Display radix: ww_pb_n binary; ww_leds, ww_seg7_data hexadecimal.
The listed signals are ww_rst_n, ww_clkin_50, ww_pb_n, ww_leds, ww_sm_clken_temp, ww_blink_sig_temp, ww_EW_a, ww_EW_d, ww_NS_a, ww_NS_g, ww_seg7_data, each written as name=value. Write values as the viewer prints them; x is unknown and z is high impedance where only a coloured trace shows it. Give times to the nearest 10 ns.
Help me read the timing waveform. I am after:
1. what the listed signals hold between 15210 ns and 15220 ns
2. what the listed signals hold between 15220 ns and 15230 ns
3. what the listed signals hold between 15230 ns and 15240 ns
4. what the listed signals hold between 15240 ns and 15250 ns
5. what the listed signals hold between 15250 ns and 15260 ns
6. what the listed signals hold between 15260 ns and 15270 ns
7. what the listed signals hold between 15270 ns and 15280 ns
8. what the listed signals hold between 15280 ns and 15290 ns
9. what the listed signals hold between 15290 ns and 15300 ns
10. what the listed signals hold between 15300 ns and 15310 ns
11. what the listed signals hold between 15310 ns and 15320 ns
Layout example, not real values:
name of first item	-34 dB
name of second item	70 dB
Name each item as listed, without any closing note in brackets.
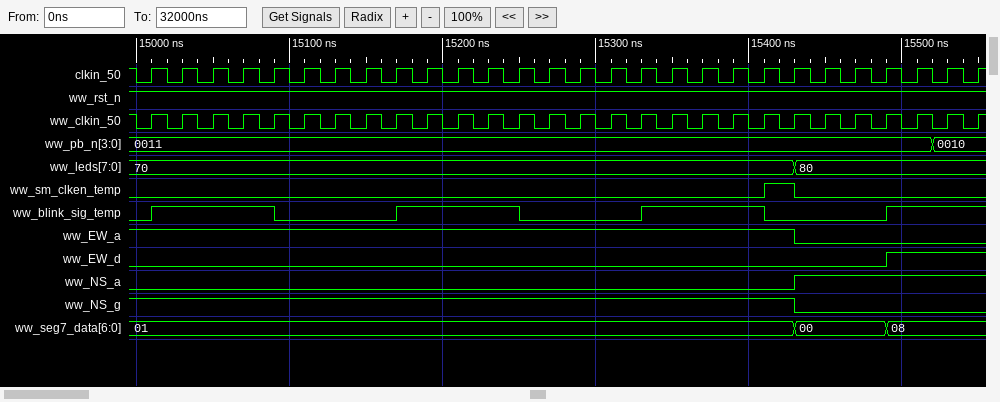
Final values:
what the listed signals hold between 15210 ns and 15220 ns	ww_rst_n=1, ww_clkin_50=1, ww_pb_n=0011, ww_leds=70, ww_sm_clken_temp=0, ww_blink_sig_temp=1, ww_EW_a=1, ww_EW_d=0, ww_NS_a=0, ww_NS_g=1, ww_seg7_data=01
what the listed signals hold between 15220 ns and 15230 ns	ww_rst_n=1, ww_clkin_50=0, ww_pb_n=0011, ww_leds=70, ww_sm_clken_temp=0, ww_blink_sig_temp=1, ww_EW_a=1, ww_EW_d=0, ww_NS_a=0, ww_NS_g=1, ww_seg7_data=01
what the listed signals hold between 15230 ns and 15240 ns	ww_rst_n=1, ww_clkin_50=1, ww_pb_n=0011, ww_leds=70, ww_sm_clken_temp=0, ww_blink_sig_temp=1, ww_EW_a=1, ww_EW_d=0, ww_NS_a=0, ww_NS_g=1, ww_seg7_data=01
what the listed signals hold between 15240 ns and 15250 ns	ww_rst_n=1, ww_clkin_50=0, ww_pb_n=0011, ww_leds=70, ww_sm_clken_temp=0, ww_blink_sig_temp=1, ww_EW_a=1, ww_EW_d=0, ww_NS_a=0, ww_NS_g=1, ww_seg7_data=01
what the listed signals hold between 15250 ns and 15260 ns	ww_rst_n=1, ww_clkin_50=1, ww_pb_n=0011, ww_leds=70, ww_sm_clken_temp=0, ww_blink_sig_temp=0, ww_EW_a=1, ww_EW_d=0, ww_NS_a=0, ww_NS_g=1, ww_seg7_data=01
what the listed signals hold between 15260 ns and 15270 ns	ww_rst_n=1, ww_clkin_50=0, ww_pb_n=0011, ww_leds=70, ww_sm_clken_temp=0, ww_blink_sig_temp=0, ww_EW_a=1, ww_EW_d=0, ww_NS_a=0, ww_NS_g=1, ww_seg7_data=01
what the listed signals hold between 15270 ns and 15280 ns	ww_rst_n=1, ww_clkin_50=1, ww_pb_n=0011, ww_leds=70, ww_sm_clken_temp=0, ww_blink_sig_temp=0, ww_EW_a=1, ww_EW_d=0, ww_NS_a=0, ww_NS_g=1, ww_seg7_data=01
what the listed signals hold between 15280 ns and 15290 ns	ww_rst_n=1, ww_clkin_50=0, ww_pb_n=0011, ww_leds=70, ww_sm_clken_temp=0, ww_blink_sig_temp=0, ww_EW_a=1, ww_EW_d=0, ww_NS_a=0, ww_NS_g=1, ww_seg7_data=01
what the listed signals hold between 15290 ns and 15300 ns	ww_rst_n=1, ww_clkin_50=1, ww_pb_n=0011, ww_leds=70, ww_sm_clken_temp=0, ww_blink_sig_temp=0, ww_EW_a=1, ww_EW_d=0, ww_NS_a=0, ww_NS_g=1, ww_seg7_data=01
what the listed signals hold between 15300 ns and 15310 ns	ww_rst_n=1, ww_clkin_50=0, ww_pb_n=0011, ww_leds=70, ww_sm_clken_temp=0, ww_blink_sig_temp=0, ww_EW_a=1, ww_EW_d=0, ww_NS_a=0, ww_NS_g=1, ww_seg7_data=01
what the listed signals hold between 15310 ns and 15320 ns	ww_rst_n=1, ww_clkin_50=1, ww_pb_n=0011, ww_leds=70, ww_sm_clken_temp=0, ww_blink_sig_temp=0, ww_EW_a=1, ww_EW_d=0, ww_NS_a=0, ww_NS_g=1, ww_seg7_data=01
